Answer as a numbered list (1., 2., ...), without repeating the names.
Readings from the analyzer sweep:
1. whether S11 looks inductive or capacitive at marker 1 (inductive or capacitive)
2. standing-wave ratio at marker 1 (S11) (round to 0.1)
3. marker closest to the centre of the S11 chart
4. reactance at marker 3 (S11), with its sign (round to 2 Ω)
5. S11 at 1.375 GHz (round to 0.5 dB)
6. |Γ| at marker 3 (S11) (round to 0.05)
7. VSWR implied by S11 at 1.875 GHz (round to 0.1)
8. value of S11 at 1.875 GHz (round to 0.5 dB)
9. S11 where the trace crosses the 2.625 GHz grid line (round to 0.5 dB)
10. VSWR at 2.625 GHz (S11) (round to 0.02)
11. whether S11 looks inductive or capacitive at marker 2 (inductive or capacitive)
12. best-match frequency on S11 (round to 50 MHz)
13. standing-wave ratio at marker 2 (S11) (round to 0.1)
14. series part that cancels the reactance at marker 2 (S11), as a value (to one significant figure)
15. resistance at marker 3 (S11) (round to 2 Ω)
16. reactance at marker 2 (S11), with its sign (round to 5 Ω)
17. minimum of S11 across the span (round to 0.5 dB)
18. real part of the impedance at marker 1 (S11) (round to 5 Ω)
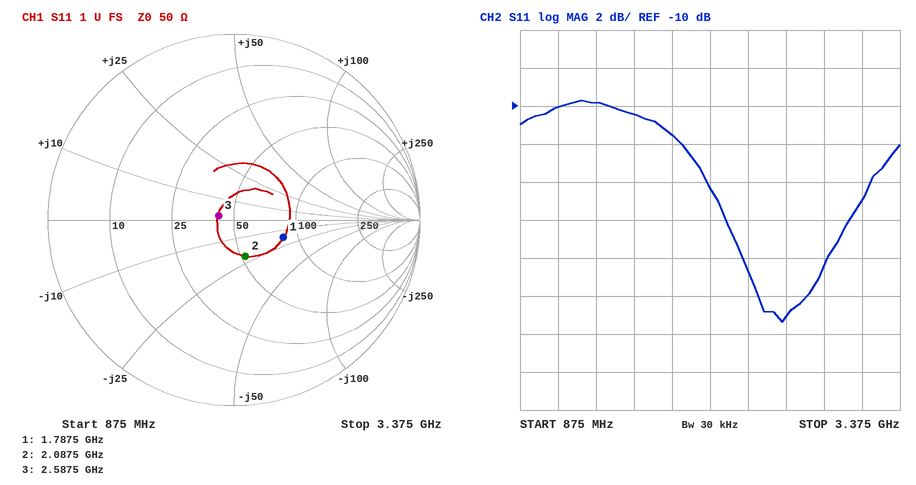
1. capacitive
2. 1.8
3. marker 3
4. +2 Ω
5. -10.0 dB
6. 0.10
7. 1.7
8. -11.5 dB
9. -21.0 dB
10. 1.20
11. capacitive
12. 2.60 GHz
13. 1.5
14. 2 nH
15. 42 Ω
16. -20 Ω
17. -21.5 dB
18. 85 Ω
